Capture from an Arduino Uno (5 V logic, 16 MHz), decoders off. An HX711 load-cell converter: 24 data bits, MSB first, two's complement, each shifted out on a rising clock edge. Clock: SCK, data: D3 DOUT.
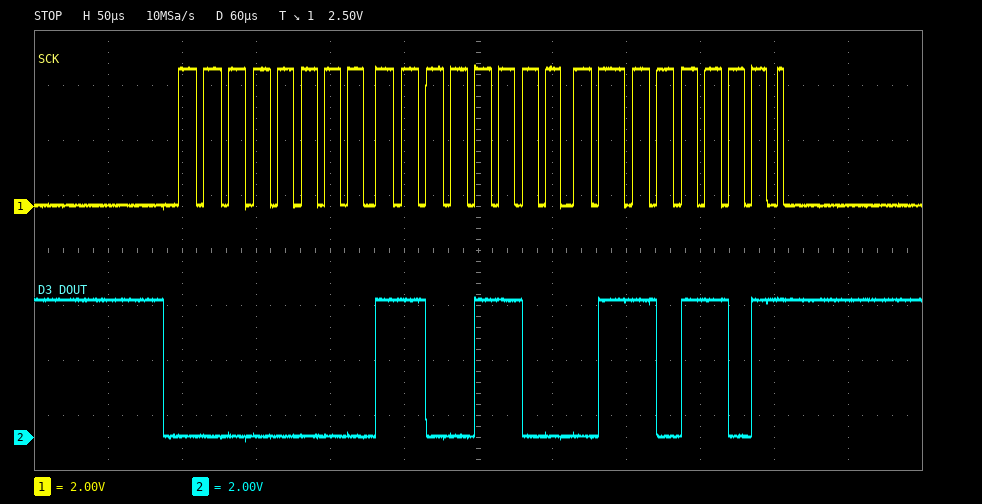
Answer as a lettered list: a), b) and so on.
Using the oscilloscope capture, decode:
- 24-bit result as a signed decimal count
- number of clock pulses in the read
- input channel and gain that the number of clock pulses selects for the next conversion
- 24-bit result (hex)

a) 52333
b) 25
c) channel A, gain 128
d) 0x00CC6D
